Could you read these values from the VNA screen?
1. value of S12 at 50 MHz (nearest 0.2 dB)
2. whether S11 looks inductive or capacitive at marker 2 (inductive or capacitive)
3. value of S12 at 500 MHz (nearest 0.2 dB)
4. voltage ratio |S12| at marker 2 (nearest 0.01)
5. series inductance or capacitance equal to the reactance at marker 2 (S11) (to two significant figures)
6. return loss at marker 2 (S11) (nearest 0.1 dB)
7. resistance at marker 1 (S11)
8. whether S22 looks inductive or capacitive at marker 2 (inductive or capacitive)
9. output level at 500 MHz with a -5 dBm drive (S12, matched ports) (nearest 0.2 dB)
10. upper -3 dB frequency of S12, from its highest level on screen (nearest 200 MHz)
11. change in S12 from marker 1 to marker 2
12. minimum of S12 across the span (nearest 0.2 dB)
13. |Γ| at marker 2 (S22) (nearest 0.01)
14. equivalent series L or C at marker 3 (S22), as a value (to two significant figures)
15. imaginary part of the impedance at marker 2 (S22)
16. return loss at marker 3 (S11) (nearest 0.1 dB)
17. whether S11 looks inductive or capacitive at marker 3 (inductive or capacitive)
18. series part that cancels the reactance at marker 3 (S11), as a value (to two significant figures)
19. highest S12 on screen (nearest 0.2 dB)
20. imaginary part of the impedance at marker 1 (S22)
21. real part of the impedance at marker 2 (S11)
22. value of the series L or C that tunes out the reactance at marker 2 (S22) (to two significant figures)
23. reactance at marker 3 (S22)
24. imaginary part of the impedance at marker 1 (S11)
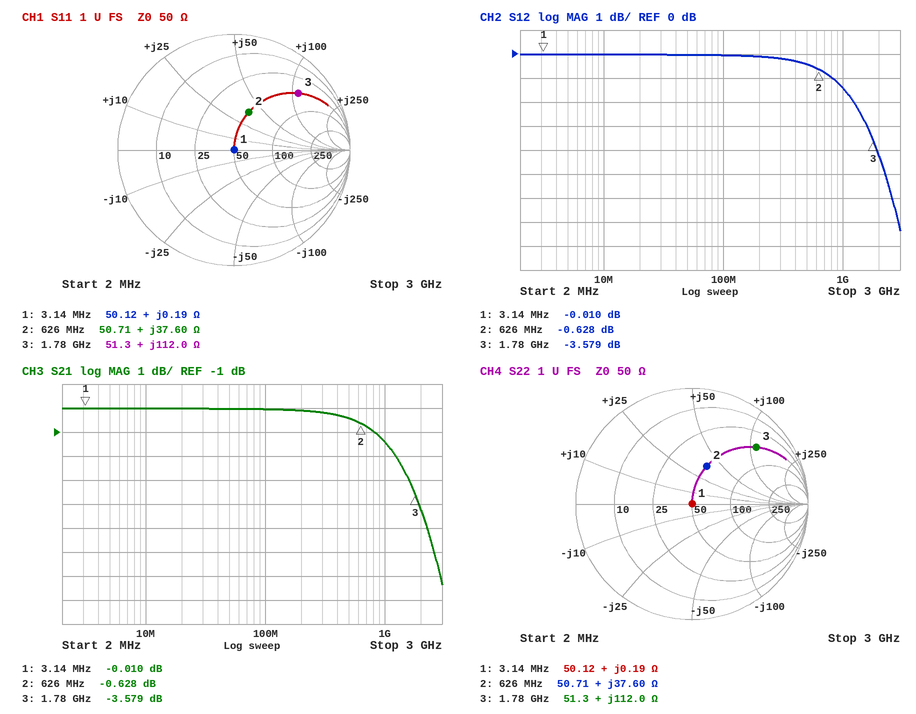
0.0 dB
inductive
-0.4 dB
0.93
9.6 nH
9.1 dB
50.12 Ω
inductive
-5.4 dBm
1.6 GHz
-0.618 dB
-7.4 dB
0.35
10 nH
+37.60 Ω
2.6 dB
inductive
800 fF
0.0 dB
+0.19 Ω
50.71 Ω
6.8 pF
+112.0 Ω
+0.19 Ω
